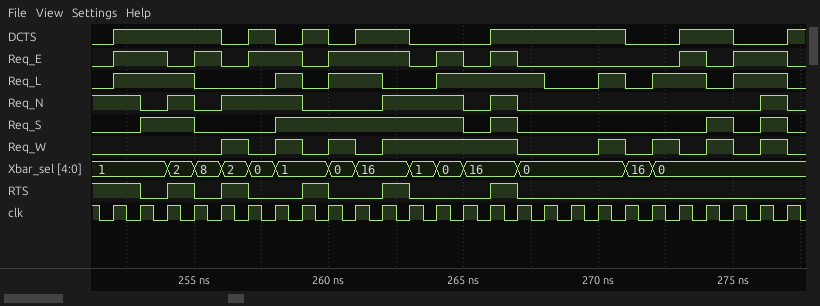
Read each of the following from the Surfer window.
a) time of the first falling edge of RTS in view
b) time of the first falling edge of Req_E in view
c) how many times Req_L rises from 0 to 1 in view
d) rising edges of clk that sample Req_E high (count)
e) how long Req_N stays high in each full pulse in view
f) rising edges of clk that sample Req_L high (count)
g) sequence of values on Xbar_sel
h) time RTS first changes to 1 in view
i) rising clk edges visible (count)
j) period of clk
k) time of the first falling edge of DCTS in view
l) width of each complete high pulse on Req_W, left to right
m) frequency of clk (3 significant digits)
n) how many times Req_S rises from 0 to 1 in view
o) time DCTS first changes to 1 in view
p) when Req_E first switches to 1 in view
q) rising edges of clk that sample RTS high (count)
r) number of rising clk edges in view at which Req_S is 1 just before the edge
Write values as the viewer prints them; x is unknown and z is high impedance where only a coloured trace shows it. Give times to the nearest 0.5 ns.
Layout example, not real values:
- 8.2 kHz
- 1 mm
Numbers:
- 253 ns
- 254 ns
- 7
- 13
- 1 ns, 3 ns, 3 ns, 1 ns, 1 ns
- 15
- 1, 2, 8, 2, 0, 1, 0, 16, 1, 0, 16, 0, 16, 0
- 254 ns
- 26
- 1 ns
- 256 ns
- 1 ns, 1 ns, 1 ns, 5 ns, 1 ns, 1 ns, 1 ns, 1 ns
- 1.00 GHz
- 5
- 252 ns
- 252 ns
- 7
- 12
